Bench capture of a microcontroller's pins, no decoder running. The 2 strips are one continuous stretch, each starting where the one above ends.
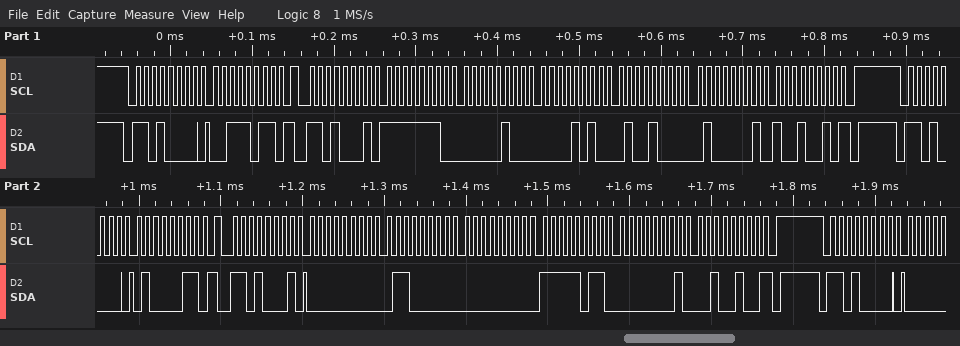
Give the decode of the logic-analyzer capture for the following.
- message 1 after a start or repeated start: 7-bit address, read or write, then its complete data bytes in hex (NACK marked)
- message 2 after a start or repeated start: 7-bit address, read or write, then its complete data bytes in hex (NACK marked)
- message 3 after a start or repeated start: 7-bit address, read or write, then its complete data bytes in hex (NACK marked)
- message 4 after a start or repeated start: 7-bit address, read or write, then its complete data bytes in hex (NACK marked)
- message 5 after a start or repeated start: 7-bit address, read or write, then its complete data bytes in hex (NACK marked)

0x68 write: 3B
0x68 read: FE 04 0A 48 41 92 NACK
0x68 write: 43
0x68 read: 00 60 00 FB 01 24 NACK
0x68 write
